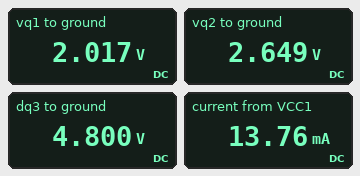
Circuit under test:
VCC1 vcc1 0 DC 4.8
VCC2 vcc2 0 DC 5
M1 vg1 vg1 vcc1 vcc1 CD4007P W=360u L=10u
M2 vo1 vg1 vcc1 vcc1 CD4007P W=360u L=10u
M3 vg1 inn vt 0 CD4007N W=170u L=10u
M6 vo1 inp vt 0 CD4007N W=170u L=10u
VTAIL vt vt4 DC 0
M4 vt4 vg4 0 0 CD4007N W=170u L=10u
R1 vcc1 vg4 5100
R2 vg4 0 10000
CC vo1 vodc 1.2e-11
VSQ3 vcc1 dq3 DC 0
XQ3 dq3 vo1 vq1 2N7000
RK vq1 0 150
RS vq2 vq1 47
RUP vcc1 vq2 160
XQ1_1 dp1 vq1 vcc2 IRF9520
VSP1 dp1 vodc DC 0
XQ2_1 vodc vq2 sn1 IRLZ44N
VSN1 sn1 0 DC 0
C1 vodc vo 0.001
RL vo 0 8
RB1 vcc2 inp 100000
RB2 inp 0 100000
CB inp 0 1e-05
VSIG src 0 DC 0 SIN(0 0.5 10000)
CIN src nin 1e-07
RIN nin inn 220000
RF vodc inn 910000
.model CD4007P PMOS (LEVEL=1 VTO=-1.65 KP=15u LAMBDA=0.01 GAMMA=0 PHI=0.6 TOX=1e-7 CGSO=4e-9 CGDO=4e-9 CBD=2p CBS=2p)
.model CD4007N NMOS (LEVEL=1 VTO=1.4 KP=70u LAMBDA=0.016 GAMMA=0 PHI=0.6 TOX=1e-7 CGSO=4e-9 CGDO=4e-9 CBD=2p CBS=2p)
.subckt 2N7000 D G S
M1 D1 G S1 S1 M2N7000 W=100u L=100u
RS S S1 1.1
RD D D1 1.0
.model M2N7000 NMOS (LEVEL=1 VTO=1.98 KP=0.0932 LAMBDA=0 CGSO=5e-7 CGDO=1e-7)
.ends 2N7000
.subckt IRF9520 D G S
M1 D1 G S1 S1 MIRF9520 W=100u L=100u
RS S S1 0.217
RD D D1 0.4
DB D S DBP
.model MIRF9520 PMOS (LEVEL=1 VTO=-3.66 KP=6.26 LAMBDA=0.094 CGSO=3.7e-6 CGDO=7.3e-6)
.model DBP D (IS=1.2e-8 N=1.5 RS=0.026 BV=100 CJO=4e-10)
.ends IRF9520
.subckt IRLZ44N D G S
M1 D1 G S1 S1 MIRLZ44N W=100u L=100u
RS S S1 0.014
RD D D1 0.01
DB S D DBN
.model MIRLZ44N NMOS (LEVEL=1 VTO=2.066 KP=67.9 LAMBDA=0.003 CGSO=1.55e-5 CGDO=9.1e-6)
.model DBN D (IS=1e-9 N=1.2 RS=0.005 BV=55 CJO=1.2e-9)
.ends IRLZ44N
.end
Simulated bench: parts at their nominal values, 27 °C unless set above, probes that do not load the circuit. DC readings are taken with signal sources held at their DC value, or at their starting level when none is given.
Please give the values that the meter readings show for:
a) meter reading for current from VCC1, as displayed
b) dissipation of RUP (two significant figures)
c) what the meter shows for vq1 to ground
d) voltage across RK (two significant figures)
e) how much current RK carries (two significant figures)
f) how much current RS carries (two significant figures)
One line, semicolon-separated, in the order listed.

13.76 mA; 29 mW; 2.017 V; 2.0 V; 13 mA; 13 mA
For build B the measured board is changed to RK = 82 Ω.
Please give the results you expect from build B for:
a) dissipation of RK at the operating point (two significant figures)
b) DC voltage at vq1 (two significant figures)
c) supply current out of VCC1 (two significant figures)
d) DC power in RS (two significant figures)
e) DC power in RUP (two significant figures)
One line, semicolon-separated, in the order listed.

23 mW; 1.4 V; 17 mA; 13 mW; 44 mW
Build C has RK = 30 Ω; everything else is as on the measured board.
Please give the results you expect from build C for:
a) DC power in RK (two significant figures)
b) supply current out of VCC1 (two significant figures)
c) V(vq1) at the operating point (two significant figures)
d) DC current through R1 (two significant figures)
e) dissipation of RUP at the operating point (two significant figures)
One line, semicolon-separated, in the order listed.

55 mW; 44 mA; 1.3 V; 320 µA; 46 mW
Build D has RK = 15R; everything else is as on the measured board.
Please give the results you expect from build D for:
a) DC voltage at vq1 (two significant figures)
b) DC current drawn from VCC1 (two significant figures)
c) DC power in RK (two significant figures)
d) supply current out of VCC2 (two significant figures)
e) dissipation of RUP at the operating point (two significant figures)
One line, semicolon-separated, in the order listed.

1.3 V; 87 mA; 110 mW; 10 mA; 46 mW
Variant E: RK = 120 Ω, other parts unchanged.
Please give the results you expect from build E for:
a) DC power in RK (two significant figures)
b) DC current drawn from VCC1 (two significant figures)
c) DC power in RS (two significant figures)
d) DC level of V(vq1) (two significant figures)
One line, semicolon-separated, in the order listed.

26 mW; 15 mA; 10 mW; 1.8 V
